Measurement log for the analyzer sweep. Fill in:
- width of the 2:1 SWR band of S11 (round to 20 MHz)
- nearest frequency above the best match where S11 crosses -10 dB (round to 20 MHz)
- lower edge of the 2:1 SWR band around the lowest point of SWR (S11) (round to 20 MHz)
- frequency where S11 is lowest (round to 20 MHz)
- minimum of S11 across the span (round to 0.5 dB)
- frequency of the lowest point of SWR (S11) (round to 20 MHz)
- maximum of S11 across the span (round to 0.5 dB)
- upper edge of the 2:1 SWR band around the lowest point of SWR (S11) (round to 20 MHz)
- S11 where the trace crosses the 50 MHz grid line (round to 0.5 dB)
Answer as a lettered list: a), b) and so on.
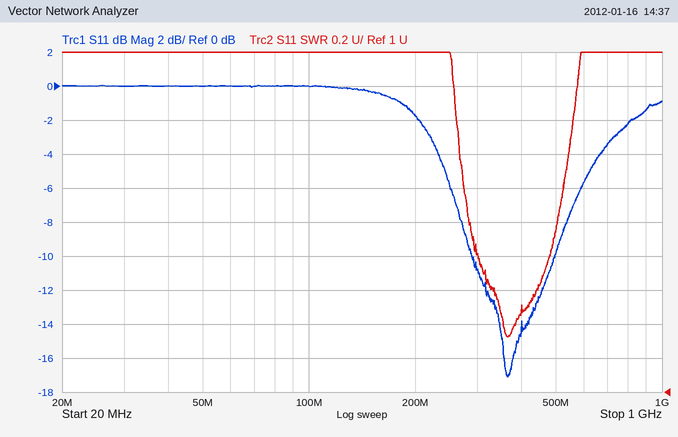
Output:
a) 220 MHz
b) 500 MHz
c) 280 MHz
d) 360 MHz
e) -17.0 dB
f) 360 MHz
g) 0.0 dB
h) 500 MHz
i) 0.0 dB
